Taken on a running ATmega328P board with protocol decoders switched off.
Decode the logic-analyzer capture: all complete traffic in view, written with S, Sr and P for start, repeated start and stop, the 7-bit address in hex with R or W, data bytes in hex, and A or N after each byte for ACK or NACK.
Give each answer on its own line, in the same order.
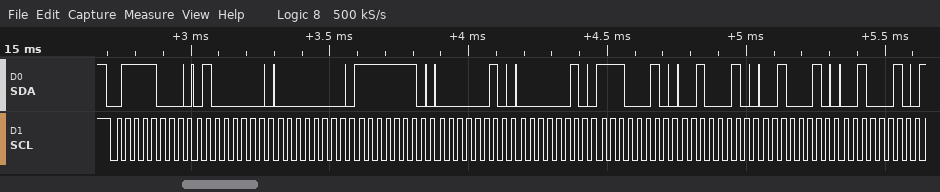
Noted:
S 3CW A 40 A 00 A FE A 02 A 02 A E2 A 22 A 22 A 22 A
